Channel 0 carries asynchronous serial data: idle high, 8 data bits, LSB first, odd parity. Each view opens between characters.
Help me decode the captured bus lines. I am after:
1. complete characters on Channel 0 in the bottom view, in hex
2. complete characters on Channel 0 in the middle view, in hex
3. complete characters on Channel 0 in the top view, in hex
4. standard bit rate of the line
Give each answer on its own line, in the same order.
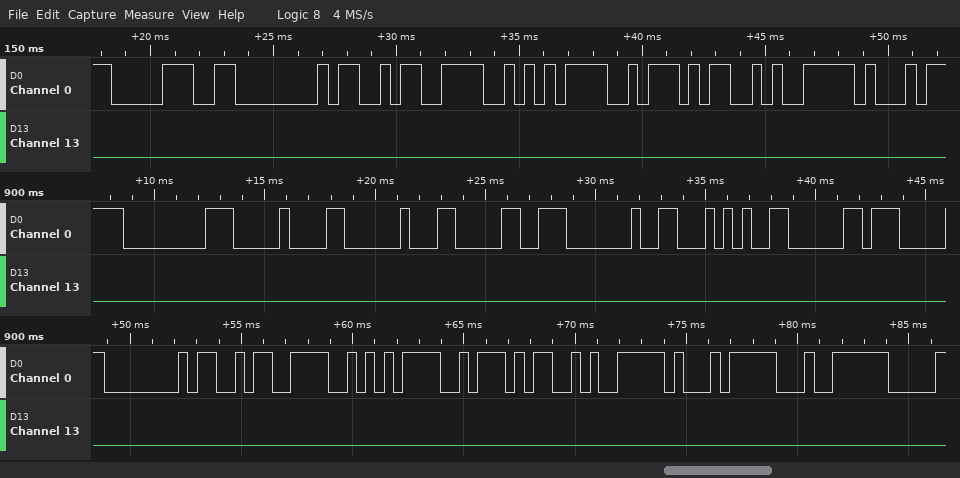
80, 9A, AA, BA, CA, D1, E4
00, 10, 20, 30, 40, 54, 60
70, 80, 9A, AA, BA, CA
2400 baud
